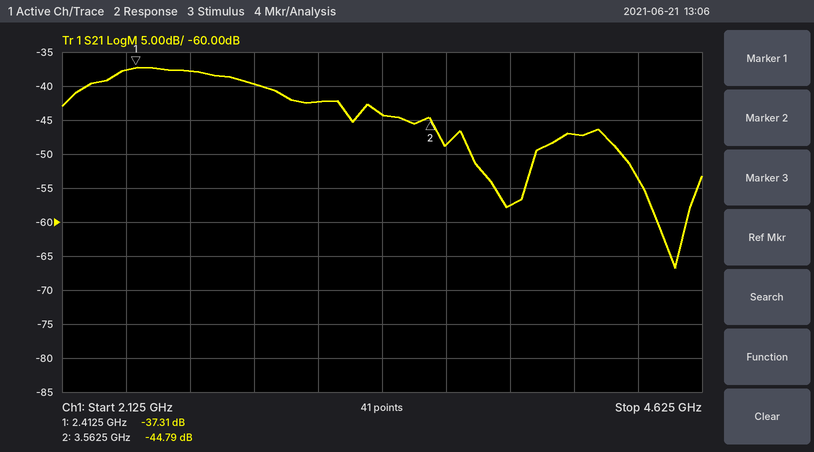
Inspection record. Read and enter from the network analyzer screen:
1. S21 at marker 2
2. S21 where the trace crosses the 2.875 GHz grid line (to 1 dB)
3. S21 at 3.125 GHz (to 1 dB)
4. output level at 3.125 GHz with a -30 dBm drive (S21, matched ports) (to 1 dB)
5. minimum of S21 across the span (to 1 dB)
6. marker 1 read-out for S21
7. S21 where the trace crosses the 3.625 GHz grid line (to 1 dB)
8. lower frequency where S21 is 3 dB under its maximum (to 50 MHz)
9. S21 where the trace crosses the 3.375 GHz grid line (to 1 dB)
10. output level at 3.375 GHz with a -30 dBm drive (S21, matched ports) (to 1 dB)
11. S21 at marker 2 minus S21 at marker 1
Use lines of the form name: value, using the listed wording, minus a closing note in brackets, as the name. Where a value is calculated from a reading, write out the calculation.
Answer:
S21 at marker 2: -44.79 dB
S21 where the trace crosses the 2.875 GHz grid line: -40 dB
S21 at 3.125 GHz: -42 dB
output level at 3.125 GHz with a -30 dBm drive (S21, matched ports): -30 dBm + (-42 dB) = -72 dBm
minimum of S21 across the span: -67 dB
marker 1 read-out for S21: -37.31 dB
S21 where the trace crosses the 3.625 GHz grid line: -49 dB
lower frequency where S21 is 3 dB under its maximum: 2.20 GHz
S21 where the trace crosses the 3.375 GHz grid line: -44 dB
output level at 3.375 GHz with a -30 dBm drive (S21, matched ports): -30 dBm + (-44 dB) = -74 dBm
S21 at marker 2 minus S21 at marker 1: -44.79 − (-37.31) = -7.48 dB
